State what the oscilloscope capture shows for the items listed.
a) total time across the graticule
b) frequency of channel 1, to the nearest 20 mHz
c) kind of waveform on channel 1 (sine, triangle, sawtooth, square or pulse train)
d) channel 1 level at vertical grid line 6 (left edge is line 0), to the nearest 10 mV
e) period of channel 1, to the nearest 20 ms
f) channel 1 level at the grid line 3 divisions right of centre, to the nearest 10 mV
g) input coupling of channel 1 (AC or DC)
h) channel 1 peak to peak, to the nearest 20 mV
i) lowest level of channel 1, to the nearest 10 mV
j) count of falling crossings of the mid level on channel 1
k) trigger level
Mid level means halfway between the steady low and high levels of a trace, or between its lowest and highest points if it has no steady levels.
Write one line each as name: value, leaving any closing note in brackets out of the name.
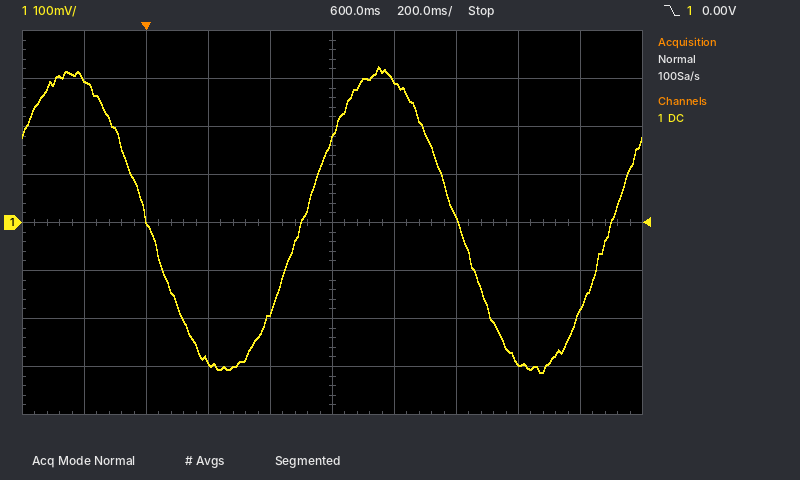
total time across the graticule: 2 s
frequency of channel 1, to the nearest 20 mHz: 1.00 Hz
kind of waveform on channel 1: sine
channel 1 level at vertical grid line 6 (left edge is line 0), to the nearest 10 mV: 300 mV
period of channel 1, to the nearest 20 ms: 1.00 s
channel 1 level at the grid line 3 divisions right of centre, to the nearest 10 mV: -290 mV
input coupling of channel 1: DC
channel 1 peak to peak, to the nearest 20 mV: 640 mV
lowest level of channel 1, to the nearest 10 mV: -310 mV
count of falling crossings of the mid level on channel 1: 2
trigger level: 0.00 V
